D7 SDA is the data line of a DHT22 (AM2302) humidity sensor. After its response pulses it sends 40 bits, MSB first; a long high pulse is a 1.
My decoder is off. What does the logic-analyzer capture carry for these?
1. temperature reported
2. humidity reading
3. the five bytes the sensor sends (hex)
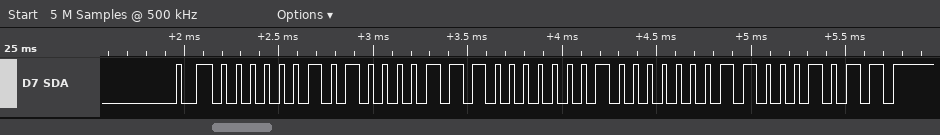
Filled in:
25.7 °C
64.7 %
02 87 01 01 8B
